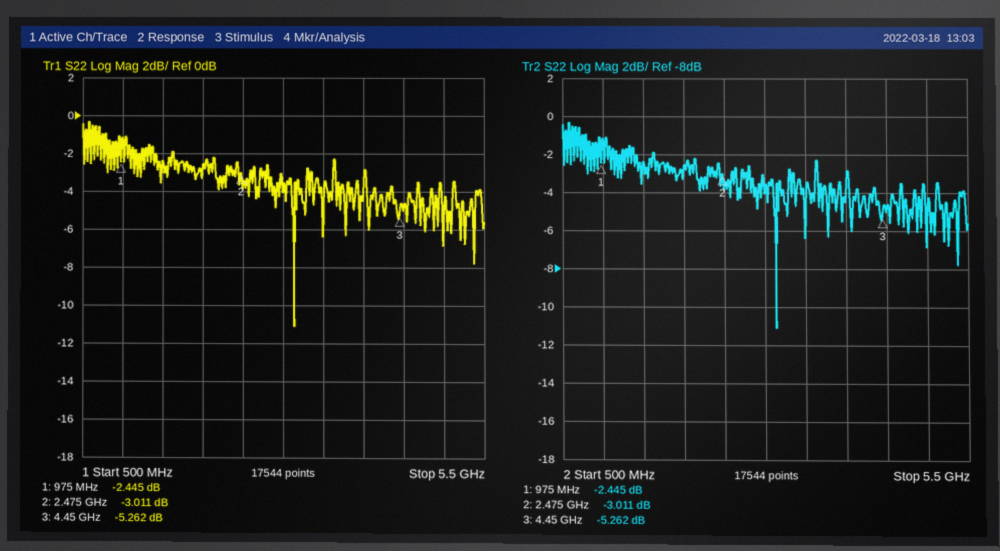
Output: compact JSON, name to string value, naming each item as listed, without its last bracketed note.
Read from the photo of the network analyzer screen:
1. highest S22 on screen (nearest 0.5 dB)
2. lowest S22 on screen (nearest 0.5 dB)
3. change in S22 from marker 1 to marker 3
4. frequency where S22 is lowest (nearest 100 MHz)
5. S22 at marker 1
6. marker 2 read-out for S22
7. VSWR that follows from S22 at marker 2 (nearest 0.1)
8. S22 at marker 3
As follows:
{"highest S22 on screen": "-0.5 dB", "lowest S22 on screen": "-11.0 dB", "change in S22 from marker 1 to marker 3": "-2.817 dB", "frequency where S22 is lowest": "3.1 GHz", "S22 at marker 1": "-2.445 dB", "marker 2 read-out for S22": "-3.011 dB", "VSWR that follows from S22 at marker 2": "5.8", "S22 at marker 3": "-5.262 dB"}
